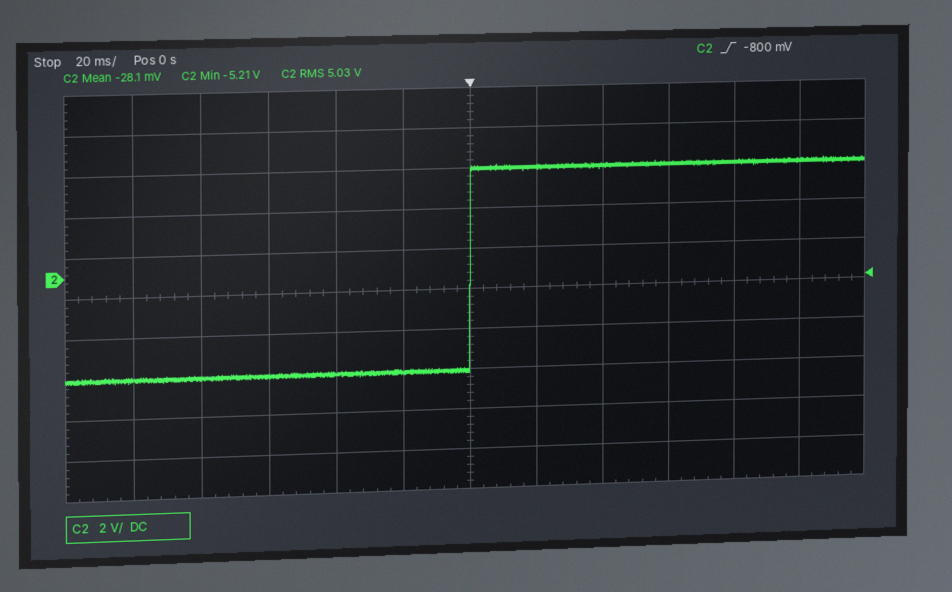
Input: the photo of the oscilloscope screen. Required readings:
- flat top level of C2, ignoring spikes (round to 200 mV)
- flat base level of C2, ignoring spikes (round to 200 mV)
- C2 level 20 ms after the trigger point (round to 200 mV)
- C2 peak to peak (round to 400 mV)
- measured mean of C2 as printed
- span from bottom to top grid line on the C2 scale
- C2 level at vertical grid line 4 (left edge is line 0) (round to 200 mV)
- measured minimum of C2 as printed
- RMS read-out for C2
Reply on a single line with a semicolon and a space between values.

5.0 V; -5.0 V; 5.0 V; 10.4 V; -28.1 mV; 20 V; -5.0 V; -5.21 V; 5.03 V
